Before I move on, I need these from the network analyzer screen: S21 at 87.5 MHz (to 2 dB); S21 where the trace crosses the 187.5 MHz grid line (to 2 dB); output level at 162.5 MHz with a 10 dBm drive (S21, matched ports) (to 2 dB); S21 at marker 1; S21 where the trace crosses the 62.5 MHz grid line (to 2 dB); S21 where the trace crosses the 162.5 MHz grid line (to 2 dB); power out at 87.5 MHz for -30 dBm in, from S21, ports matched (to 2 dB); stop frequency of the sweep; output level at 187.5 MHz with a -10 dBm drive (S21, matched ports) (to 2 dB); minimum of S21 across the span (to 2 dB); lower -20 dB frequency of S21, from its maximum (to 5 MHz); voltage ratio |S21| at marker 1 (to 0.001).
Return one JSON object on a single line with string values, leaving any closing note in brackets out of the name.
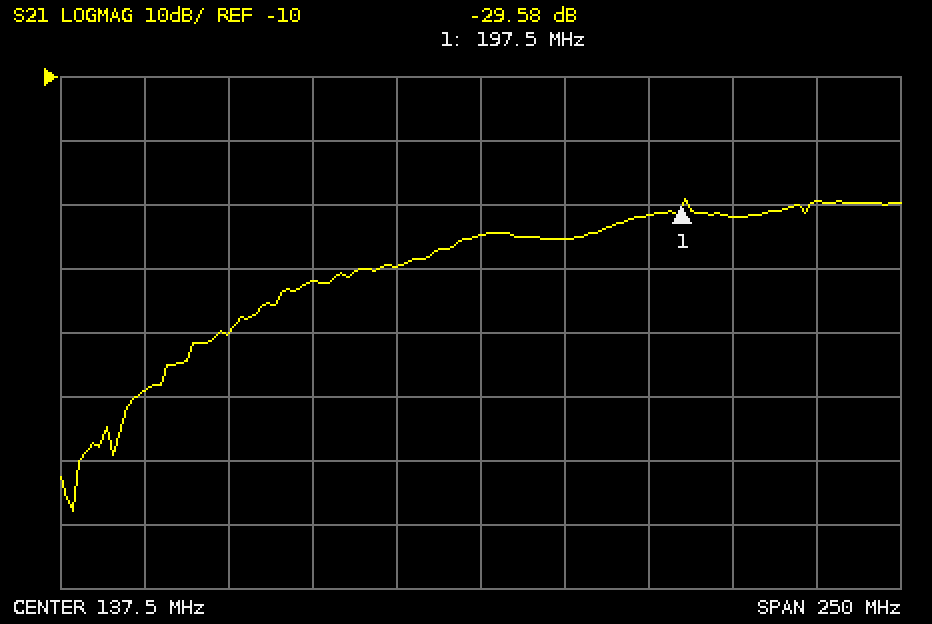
{"S21 at 87.5 MHz": "-42 dB", "S21 where the trace crosses the 187.5 MHz grid line": "-32 dB", "output level at 162.5 MHz with a 10 dBm drive (S21, matched ports)": "-26 dBm", "S21 at marker 1": "-29.58 dB", "S21 where the trace crosses the 62.5 MHz grid line": "-50 dB", "S21 where the trace crosses the 162.5 MHz grid line": "-36 dB", "power out at 87.5 MHz for -30 dBm in, from S21, ports matched": "-72 dBm", "stop frequency of the sweep": "262.5 MHz", "output level at 187.5 MHz with a -10 dBm drive (S21, matched ports)": "-42 dBm", "minimum of S21 across the span": "-78 dB", "lower -20 dB frequency of S21, from its maximum": "65 MHz", "voltage ratio |S21| at marker 1": "0.033"}
